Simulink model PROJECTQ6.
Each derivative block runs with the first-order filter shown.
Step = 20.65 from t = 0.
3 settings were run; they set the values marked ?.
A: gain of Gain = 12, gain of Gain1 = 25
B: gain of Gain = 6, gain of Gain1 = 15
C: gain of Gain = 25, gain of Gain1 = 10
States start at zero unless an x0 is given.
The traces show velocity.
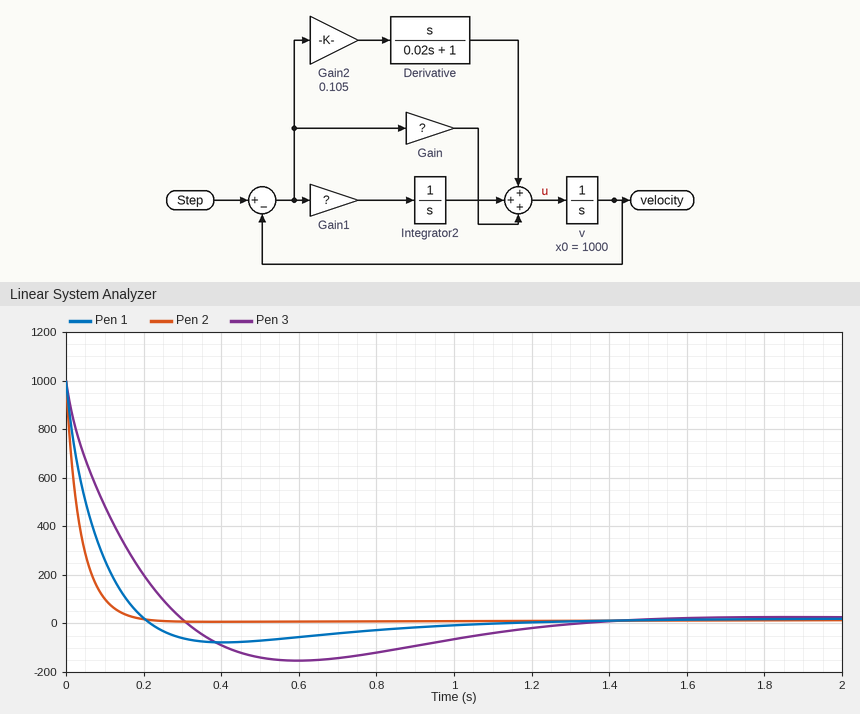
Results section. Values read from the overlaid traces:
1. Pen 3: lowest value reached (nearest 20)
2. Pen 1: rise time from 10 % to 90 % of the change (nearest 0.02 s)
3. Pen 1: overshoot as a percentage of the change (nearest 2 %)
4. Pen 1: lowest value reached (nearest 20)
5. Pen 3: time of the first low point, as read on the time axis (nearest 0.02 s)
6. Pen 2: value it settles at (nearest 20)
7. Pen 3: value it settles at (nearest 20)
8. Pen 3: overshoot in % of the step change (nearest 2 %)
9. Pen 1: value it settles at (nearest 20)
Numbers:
-160
0.14 s
10 %
-80
0.60 s
20
20
18 %
20
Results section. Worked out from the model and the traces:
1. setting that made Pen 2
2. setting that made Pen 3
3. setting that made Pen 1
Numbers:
C
B
A
